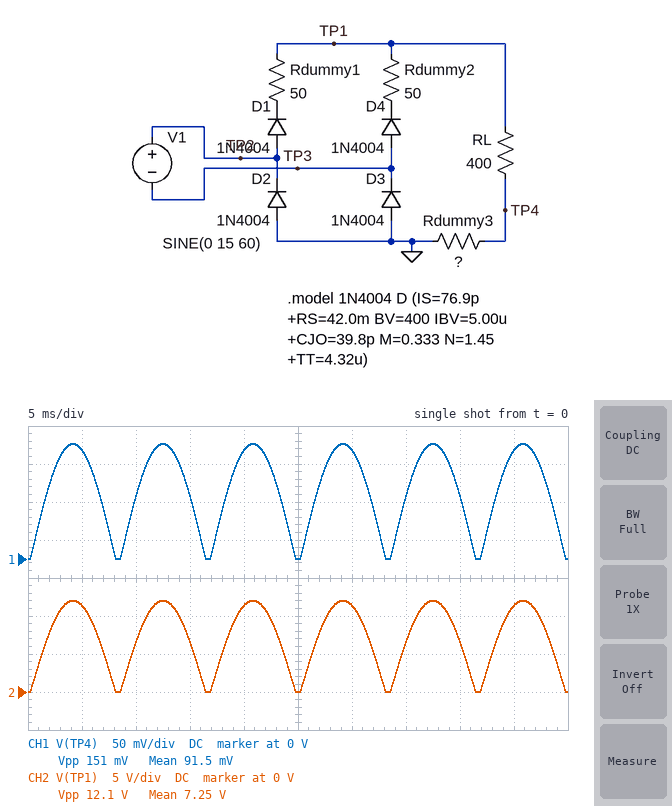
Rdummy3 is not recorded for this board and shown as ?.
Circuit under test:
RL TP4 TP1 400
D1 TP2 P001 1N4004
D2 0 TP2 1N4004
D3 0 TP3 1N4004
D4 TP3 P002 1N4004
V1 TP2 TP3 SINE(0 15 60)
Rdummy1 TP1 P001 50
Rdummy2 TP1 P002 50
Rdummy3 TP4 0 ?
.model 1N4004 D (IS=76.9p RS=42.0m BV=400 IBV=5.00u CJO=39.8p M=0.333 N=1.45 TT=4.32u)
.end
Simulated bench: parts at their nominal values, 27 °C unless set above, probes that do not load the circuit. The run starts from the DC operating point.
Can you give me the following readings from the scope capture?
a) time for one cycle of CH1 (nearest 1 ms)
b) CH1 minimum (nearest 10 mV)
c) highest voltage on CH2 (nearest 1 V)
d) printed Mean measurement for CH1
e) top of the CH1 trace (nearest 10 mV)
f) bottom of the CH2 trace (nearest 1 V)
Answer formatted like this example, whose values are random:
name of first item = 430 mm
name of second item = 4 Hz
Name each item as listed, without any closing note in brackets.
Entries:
time for one cycle of CH1 = 8 ms
CH1 minimum = 0 V
highest voltage on CH2 = 12 V
printed Mean measurement for CH1 = 91.5 mV
top of the CH1 trace = 150 mV
bottom of the CH2 trace = 0 V
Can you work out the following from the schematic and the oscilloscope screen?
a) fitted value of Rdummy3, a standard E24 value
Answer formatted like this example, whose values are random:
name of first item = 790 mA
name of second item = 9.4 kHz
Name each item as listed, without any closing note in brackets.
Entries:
fitted value of Rdummy3, a standard E24 value = 5.1 Ω
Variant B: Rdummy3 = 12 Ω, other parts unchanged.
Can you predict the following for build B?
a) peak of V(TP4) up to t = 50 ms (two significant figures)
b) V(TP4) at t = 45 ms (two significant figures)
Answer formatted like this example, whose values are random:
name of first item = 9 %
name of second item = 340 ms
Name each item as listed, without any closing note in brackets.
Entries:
peak of V(TP4) up to t = 50 ms = 350 mV
V(TP4) at t = 45 ms = 330 mV
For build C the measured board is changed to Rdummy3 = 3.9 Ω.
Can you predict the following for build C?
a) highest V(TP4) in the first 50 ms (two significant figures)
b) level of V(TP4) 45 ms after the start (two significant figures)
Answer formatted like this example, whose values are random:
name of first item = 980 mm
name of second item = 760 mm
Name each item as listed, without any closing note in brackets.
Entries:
highest V(TP4) in the first 50 ms = 120 mV
level of V(TP4) 45 ms after the start = 110 mV
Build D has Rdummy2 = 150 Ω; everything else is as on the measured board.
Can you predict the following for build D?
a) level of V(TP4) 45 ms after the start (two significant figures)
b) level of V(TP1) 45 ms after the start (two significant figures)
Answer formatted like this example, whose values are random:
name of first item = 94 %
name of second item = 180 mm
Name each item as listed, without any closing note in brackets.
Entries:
level of V(TP4) 45 ms after the start = 120 mV
level of V(TP1) 45 ms after the start = 9.3 V
